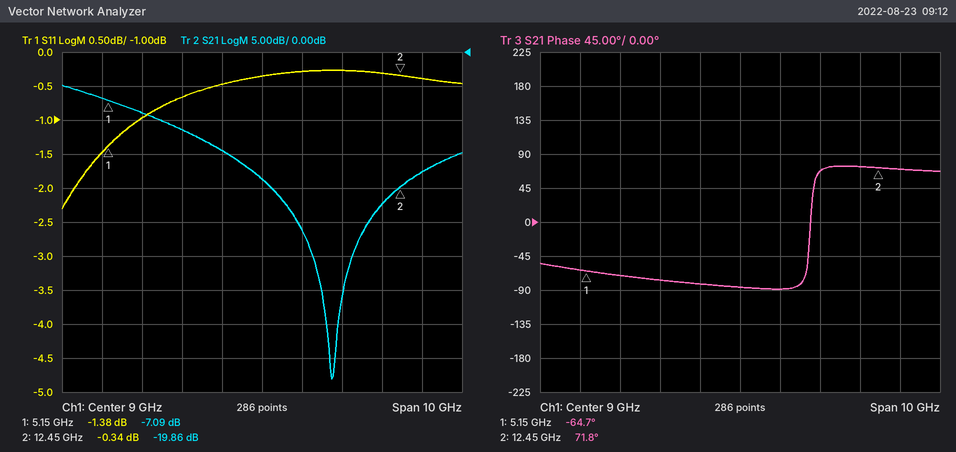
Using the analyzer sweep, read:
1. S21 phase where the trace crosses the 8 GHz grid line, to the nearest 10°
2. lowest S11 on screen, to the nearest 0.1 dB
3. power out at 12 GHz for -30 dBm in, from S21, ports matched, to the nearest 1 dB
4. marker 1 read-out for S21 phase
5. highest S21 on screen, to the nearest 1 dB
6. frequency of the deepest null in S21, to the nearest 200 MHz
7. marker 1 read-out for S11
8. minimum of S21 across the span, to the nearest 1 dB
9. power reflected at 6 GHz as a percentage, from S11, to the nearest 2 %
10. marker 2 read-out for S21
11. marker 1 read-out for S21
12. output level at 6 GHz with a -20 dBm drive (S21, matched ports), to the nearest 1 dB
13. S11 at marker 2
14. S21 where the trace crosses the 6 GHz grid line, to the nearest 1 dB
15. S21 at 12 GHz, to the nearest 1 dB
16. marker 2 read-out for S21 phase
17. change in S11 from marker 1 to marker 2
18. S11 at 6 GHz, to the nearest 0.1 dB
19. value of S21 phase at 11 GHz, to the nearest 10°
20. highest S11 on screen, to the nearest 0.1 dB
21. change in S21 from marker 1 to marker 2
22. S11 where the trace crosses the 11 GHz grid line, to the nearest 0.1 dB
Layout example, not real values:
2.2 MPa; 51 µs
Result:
-80°; -2.3 dB; -52 dBm; -64.7°; -5 dB; 10.8 GHz; -1.38 dB; -48 dB; 80 %; -19.86 dB; -7.09 dB; -29 dBm; -0.34 dB; -9 dB; -22 dB; 71.8°; 1.04 dB; -1.0 dB; 70°; -0.3 dB; -12.77 dB; -0.3 dB
